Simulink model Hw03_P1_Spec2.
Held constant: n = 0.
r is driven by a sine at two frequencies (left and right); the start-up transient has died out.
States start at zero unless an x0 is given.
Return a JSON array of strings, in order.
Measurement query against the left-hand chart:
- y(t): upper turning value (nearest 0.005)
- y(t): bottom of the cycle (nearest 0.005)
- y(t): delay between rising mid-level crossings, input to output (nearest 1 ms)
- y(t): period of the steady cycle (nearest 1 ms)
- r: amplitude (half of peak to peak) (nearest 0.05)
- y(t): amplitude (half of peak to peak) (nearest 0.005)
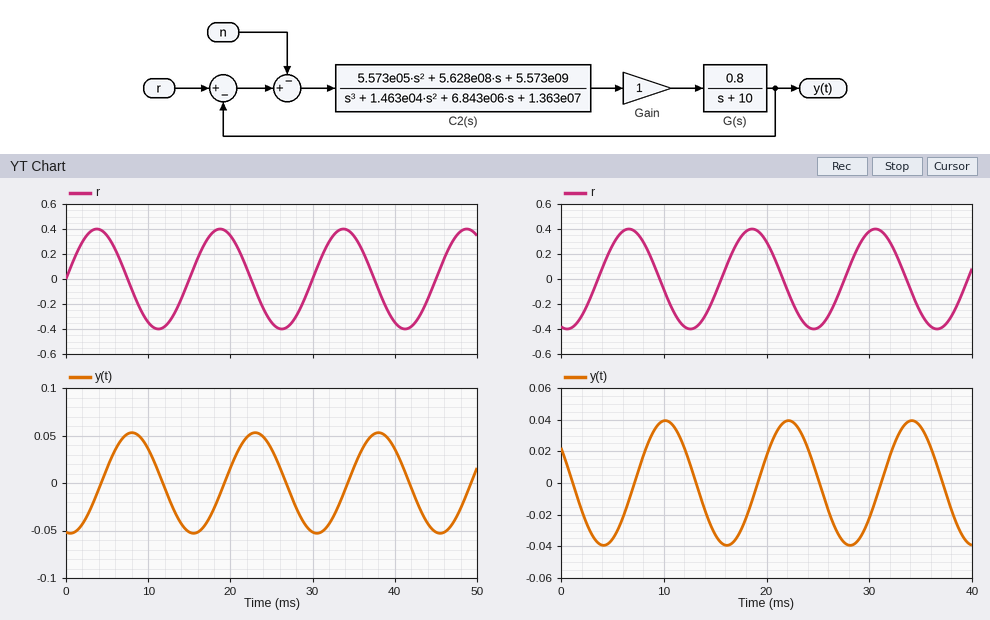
["0.055", "-0.055", "4 ms", "15 ms", "0.40", "0.055"]
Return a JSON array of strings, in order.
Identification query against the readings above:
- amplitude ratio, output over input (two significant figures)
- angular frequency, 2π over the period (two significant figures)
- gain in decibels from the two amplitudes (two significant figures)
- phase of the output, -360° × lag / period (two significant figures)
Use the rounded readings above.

["0.14", "0.42 rad/ms", "-17 dB", "-96°"]
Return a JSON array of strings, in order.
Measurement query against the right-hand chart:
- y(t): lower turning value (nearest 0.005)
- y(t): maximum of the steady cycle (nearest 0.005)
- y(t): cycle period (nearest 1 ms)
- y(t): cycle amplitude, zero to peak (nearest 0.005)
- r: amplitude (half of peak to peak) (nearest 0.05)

["-0.040", "0.040", "12 ms", "0.040", "0.40"]
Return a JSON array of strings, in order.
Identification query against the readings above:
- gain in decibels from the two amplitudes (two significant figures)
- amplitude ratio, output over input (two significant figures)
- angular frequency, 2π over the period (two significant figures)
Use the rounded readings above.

["-20 dB", "0.10", "0.52 rad/ms"]
